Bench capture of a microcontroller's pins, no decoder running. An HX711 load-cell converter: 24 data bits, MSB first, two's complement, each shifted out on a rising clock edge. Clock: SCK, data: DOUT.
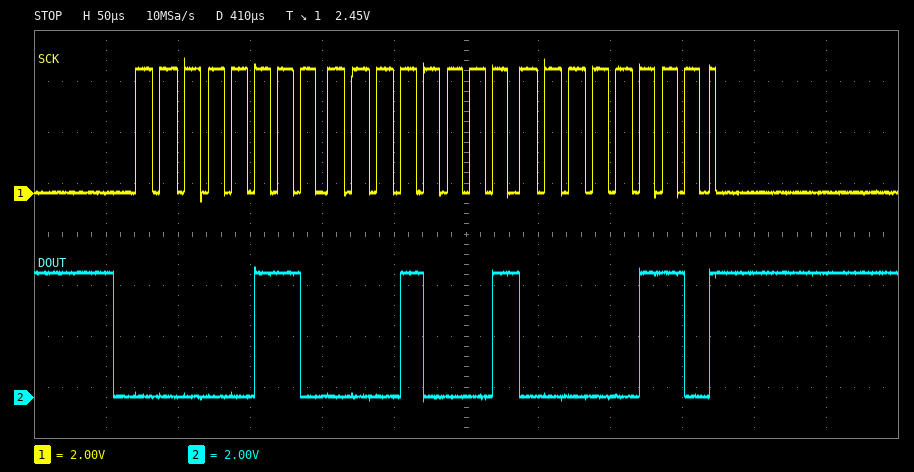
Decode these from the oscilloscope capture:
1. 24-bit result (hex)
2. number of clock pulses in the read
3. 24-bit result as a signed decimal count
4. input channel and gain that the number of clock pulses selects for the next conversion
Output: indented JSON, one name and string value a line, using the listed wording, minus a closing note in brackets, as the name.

{
  "24-bit result": "0x061106",
  "number of clock pulses in the read": "25",
  "24-bit result as a signed decimal count": "397574",
  "input channel and gain that the number of clock pulses selects for the next conversion": "channel A, gain 128"
}
